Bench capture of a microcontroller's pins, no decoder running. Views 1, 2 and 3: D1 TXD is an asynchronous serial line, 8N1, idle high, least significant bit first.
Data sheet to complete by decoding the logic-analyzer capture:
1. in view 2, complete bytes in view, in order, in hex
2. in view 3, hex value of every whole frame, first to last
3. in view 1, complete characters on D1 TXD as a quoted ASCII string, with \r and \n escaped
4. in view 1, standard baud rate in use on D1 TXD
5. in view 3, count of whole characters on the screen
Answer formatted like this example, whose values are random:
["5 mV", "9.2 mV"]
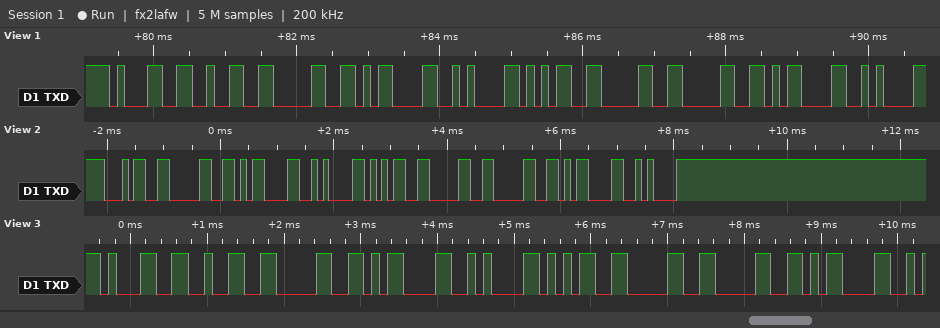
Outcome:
["34 30 0D 0A 35 30 30 0D 0A", "31 32 30 0D 0A 35 30 30 0D", "\"120\\r\\n500\\r\\n\"", "9600 baud", "9"]
